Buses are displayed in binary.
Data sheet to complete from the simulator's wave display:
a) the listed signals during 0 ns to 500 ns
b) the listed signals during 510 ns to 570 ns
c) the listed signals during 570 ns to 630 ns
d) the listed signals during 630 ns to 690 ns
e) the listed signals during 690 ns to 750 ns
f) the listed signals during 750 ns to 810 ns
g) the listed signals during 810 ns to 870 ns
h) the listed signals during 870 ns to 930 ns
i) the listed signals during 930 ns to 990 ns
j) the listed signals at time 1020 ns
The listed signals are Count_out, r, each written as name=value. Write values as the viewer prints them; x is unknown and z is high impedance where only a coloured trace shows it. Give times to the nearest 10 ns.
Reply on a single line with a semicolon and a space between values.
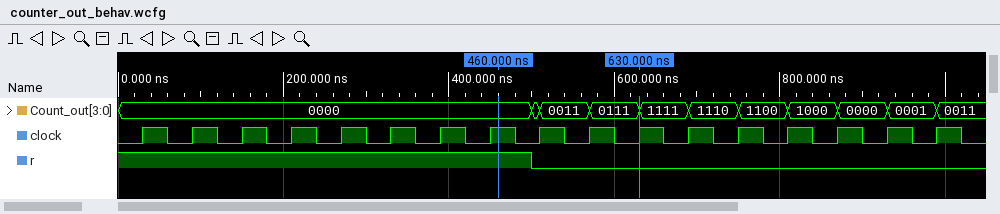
Count_out=0000, r=1; Count_out=0011, r=0; Count_out=0111, r=0; Count_out=1111, r=0; Count_out=1110, r=0; Count_out=1100, r=0; Count_out=1000, r=0; Count_out=0000, r=0; Count_out=0001, r=0; Count_out=0011, r=0
